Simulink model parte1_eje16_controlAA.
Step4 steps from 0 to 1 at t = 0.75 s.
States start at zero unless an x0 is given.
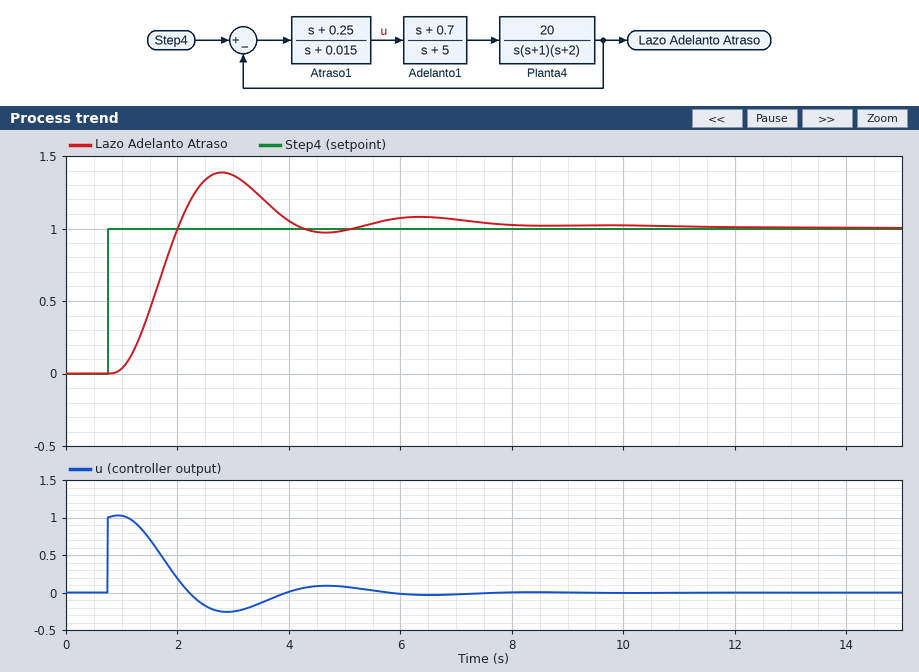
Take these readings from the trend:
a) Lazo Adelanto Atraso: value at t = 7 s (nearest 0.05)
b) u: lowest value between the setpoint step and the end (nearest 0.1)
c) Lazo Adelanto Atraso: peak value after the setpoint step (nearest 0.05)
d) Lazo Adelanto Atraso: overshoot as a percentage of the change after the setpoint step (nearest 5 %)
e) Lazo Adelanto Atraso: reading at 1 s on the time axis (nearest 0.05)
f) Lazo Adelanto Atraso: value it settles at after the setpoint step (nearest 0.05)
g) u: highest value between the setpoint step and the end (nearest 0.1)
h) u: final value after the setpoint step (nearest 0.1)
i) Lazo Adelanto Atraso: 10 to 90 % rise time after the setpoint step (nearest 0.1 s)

1.05
-0.3
1.40
40 %
0.05
1.00
1.0
0.0
0.8 s
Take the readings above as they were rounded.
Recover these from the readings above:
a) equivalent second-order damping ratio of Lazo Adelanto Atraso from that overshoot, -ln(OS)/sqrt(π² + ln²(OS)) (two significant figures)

0.28
